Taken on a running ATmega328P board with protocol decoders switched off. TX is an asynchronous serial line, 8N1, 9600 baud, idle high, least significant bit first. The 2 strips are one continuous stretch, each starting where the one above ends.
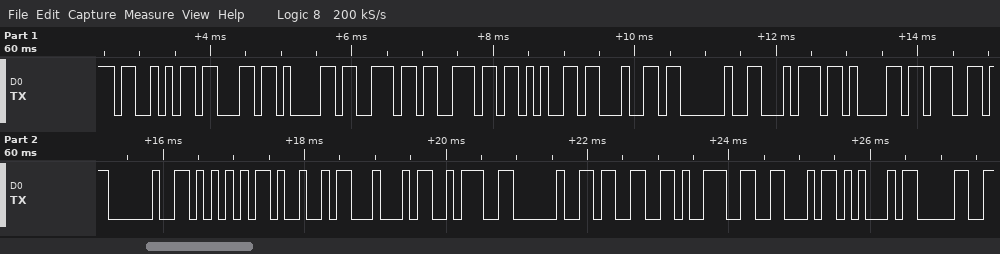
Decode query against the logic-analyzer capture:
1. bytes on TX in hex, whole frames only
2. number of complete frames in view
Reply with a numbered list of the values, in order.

1. 53 63 61 6E 6E 65 64 20 74 61 67 20 55 49 44 3A 20 33 39 46 45 30
2. 22
